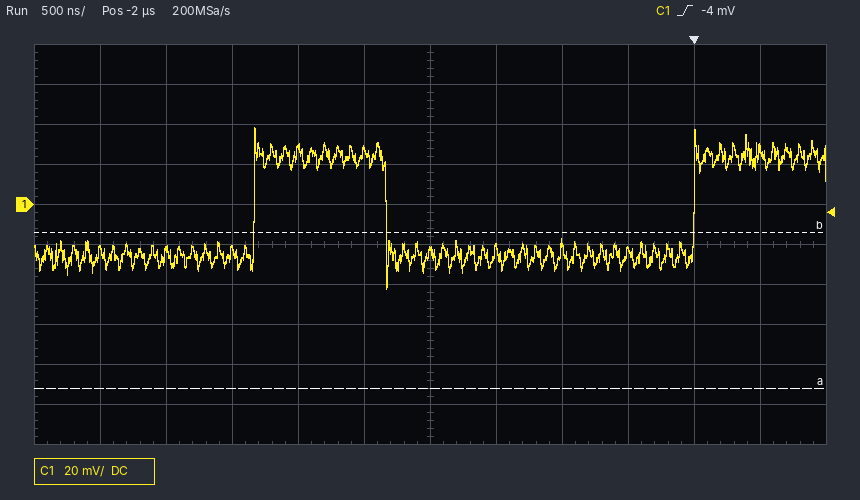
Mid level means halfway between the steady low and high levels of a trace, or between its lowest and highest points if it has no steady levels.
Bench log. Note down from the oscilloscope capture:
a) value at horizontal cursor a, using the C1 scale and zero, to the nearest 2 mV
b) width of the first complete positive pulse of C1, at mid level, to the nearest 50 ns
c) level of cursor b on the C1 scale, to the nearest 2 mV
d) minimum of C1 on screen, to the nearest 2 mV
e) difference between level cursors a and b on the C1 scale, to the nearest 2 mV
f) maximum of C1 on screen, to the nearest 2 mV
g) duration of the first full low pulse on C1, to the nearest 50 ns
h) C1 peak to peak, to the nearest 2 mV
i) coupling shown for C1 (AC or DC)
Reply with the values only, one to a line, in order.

-92 mV
1.00 µs
-14 mV
-42 mV
78 mV
38 mV
2.35 µs
80 mV
DC
